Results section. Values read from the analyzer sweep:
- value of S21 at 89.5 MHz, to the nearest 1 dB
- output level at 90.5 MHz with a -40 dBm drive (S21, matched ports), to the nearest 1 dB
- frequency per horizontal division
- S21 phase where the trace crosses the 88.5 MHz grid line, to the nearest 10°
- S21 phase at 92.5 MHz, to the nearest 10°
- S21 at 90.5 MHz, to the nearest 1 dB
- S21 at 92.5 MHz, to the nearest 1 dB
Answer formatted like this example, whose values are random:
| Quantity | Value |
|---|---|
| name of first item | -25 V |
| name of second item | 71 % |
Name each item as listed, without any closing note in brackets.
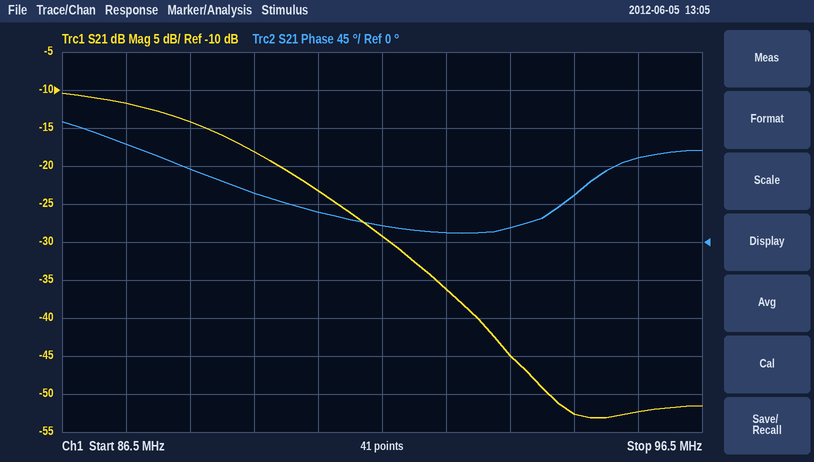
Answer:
| Quantity | Value |
|---|---|
| value of S21 at 89.5 MHz, to the nearest 1 dB | -18 dB |
| output level at 90.5 MHz with a -40 dBm drive (S21, matched ports), to the nearest 1 dB | -63 dBm |
| frequency per horizontal division | 1 MHz |
| S21 phase where the trace crosses the 88.5 MHz grid line, to the nearest 10° | 90° |
| S21 phase at 92.5 MHz, to the nearest 10° | 10° |
| S21 at 90.5 MHz, to the nearest 1 dB | -23 dB |
| S21 at 92.5 MHz, to the nearest 1 dB | -36 dB |
